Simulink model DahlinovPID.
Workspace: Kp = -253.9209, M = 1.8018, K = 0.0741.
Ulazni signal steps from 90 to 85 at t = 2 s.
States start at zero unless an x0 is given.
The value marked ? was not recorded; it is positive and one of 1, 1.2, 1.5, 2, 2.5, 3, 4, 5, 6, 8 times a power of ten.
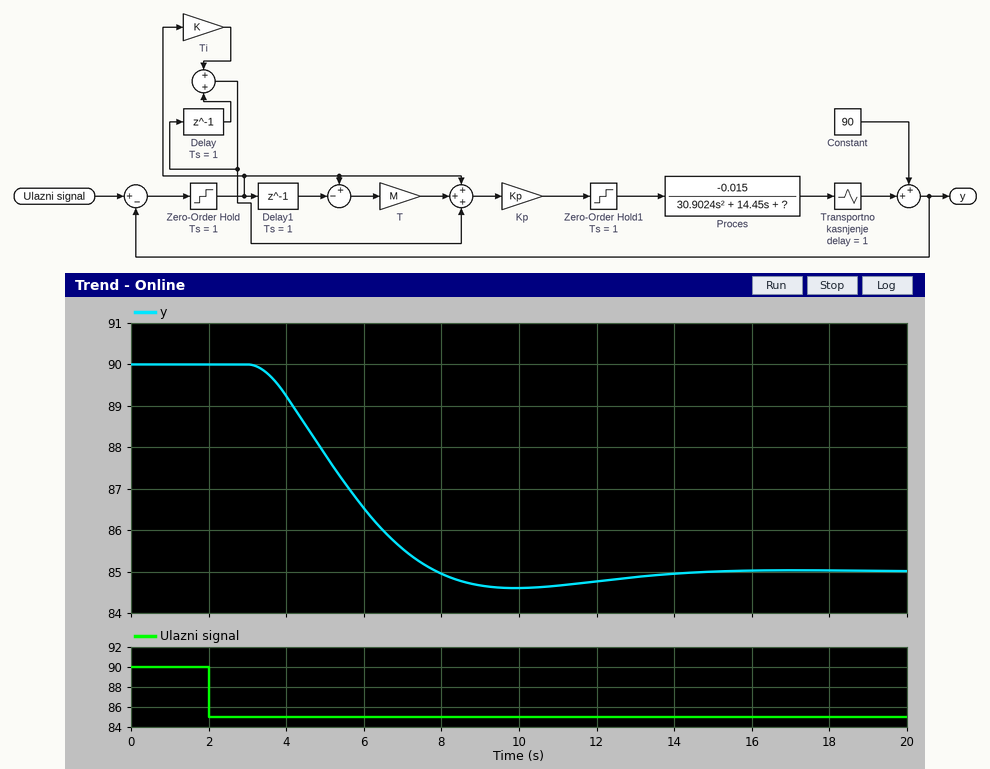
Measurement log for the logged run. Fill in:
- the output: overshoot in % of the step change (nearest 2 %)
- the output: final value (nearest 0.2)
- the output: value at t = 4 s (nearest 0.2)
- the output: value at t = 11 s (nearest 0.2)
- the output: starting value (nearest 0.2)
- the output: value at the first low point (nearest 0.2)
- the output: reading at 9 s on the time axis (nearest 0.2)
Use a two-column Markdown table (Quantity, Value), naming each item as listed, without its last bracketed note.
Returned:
| Quantity | Value |
|---|---|
| the output: overshoot in % of the step change | 8 % |
| the output: final value | 85.0 |
| the output: value at t = 4 s | 89.2 |
| the output: value at t = 11 s | 84.6 |
| the output: starting value | 90.0 |
| the output: value at the first low point | 84.6 |
| the output: reading at 9 s on the time axis | 84.6 |
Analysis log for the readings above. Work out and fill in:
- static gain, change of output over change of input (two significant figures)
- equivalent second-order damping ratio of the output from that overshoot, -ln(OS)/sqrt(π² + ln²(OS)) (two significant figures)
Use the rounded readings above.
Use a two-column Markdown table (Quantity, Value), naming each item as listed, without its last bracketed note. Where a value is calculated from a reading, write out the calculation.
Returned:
| Quantity | Value |
|---|---|
| static gain, change of output over change of input | (85 - 90) / (85 - 90) = 1.0 |
| equivalent second-order damping ratio of the output from that overshoot, -ln(OS)/sqrt(π² + ln²(OS)) | ln(0.08) = -2.526; 2.526 / sqrt(9.870 + 6.379) = 0.63 |
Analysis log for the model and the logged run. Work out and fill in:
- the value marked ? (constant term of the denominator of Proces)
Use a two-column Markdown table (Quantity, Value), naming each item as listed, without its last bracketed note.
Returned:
| Quantity | Value |
|---|---|
| the value marked ? | 1 |
